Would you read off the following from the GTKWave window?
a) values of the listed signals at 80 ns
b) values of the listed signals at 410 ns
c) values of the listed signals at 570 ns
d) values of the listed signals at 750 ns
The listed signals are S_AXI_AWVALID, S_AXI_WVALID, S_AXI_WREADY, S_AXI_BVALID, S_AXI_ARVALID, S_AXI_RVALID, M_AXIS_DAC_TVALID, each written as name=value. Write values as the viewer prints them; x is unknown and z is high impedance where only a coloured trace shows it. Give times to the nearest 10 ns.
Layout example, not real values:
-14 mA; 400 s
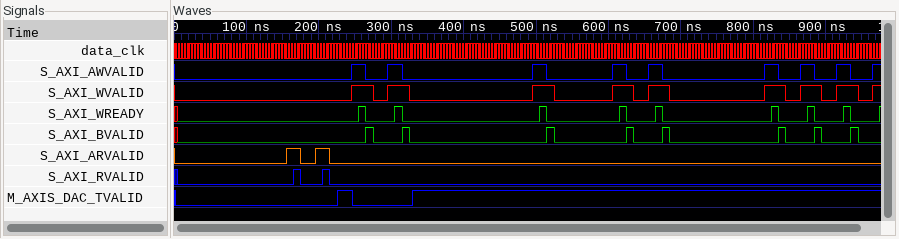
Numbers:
S_AXI_AWVALID=0, S_AXI_WVALID=0, S_AXI_WREADY=0, S_AXI_BVALID=0, S_AXI_ARVALID=0, S_AXI_RVALID=0, M_AXIS_DAC_TVALID=0; S_AXI_AWVALID=0, S_AXI_WVALID=0, S_AXI_WREADY=0, S_AXI_BVALID=0, S_AXI_ARVALID=0, S_AXI_RVALID=0, M_AXIS_DAC_TVALID=1; S_AXI_AWVALID=0, S_AXI_WVALID=0, S_AXI_WREADY=0, S_AXI_BVALID=0, S_AXI_ARVALID=0, S_AXI_RVALID=0, M_AXIS_DAC_TVALID=1; S_AXI_AWVALID=0, S_AXI_WVALID=0, S_AXI_WREADY=0, S_AXI_BVALID=0, S_AXI_ARVALID=0, S_AXI_RVALID=0, M_AXIS_DAC_TVALID=1
